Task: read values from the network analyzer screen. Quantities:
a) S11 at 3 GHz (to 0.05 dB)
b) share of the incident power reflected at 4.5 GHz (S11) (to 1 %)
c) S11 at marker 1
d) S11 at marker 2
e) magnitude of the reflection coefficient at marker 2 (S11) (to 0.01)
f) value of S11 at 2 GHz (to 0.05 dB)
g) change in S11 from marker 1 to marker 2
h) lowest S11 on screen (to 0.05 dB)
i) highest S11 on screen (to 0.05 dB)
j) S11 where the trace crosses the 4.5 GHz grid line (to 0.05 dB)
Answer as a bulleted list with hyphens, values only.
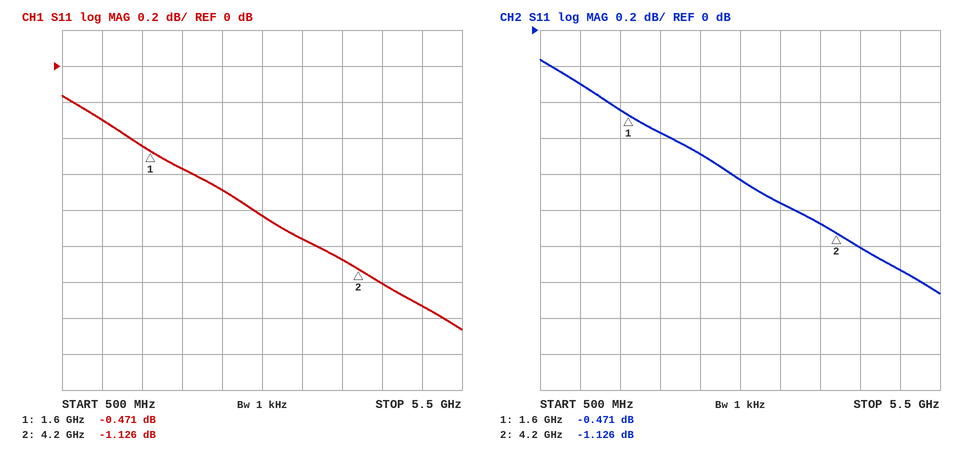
- -0.85 dB
- 76 %
- -0.471 dB
- -1.126 dB
- 0.88
- -0.55 dB
- -0.655 dB
- -1.45 dB
- -0.15 dB
- -1.20 dB
